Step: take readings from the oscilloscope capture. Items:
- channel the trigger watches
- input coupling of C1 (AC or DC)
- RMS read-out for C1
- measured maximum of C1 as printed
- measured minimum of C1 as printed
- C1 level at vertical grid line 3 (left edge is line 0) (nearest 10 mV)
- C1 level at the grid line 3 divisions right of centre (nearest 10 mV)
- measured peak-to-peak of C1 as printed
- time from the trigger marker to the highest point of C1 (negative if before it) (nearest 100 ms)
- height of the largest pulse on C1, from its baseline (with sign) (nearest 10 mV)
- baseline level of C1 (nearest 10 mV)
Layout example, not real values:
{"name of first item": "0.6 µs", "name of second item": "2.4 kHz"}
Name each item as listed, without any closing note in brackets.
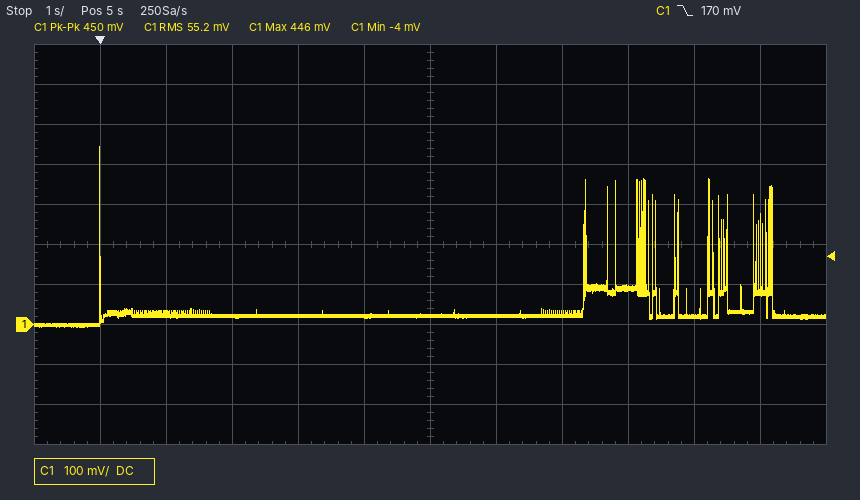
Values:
{"channel the trigger watches": "C1", "input coupling of C1": "DC", "RMS read-out for C1": "55.2 mV", "measured maximum of C1 as printed": "446 mV", "measured minimum of C1 as printed": "-4 mV", "C1 level at vertical grid line 3 (left edge is line 0)": "20 mV", "C1 level at the grid line 3 divisions right of centre": "90 mV", "measured peak-to-peak of C1 as printed": "450 mV", "time from the trigger marker to the highest point of C1 (negative if before it)": "0.0 s", "height of the largest pulse on C1, from its baseline (with sign)": "+420 mV", "baseline level of C1": "20 mV"}
